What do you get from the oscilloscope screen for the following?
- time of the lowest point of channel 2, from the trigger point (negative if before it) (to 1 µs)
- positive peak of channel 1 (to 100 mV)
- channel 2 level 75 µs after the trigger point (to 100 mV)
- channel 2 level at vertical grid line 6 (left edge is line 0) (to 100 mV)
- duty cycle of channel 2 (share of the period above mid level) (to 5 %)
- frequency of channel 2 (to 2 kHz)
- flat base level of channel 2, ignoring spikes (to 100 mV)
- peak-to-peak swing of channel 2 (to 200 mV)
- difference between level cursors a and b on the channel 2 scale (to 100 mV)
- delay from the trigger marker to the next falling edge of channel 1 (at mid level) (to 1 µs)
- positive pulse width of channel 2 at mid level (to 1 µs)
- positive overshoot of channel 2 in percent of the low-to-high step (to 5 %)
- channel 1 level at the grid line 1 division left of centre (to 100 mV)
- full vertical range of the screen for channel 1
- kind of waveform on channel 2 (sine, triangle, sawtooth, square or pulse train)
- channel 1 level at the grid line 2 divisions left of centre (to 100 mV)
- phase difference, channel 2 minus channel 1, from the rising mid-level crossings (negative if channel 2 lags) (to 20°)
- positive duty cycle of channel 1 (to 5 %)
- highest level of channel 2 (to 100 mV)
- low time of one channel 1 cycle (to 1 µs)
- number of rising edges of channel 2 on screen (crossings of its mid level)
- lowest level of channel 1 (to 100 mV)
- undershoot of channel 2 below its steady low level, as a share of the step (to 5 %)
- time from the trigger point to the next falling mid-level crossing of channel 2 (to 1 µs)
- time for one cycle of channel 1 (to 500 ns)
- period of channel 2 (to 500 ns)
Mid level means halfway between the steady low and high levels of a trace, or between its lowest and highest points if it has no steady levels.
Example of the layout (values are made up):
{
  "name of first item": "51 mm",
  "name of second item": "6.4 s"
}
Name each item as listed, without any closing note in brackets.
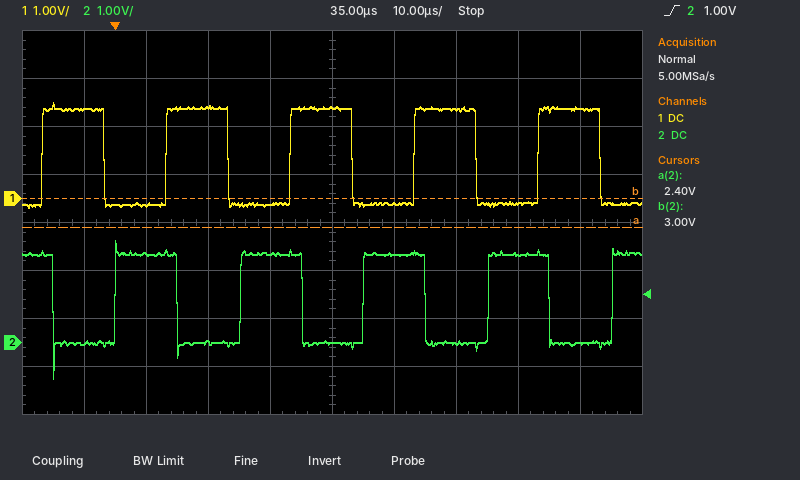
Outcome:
{
  "time of the lowest point of channel 2, from the trigger point (negative if before it)": "-10 µs",
  "positive peak of channel 1": "2.0 V",
  "channel 2 level 75 µs after the trigger point": "0.0 V",
  "channel 2 level at vertical grid line 6 (left edge is line 0)": "1.8 V",
  "duty cycle of channel 2 (share of the period above mid level)": "50 %",
  "frequency of channel 2": "50 kHz",
  "flat base level of channel 2, ignoring spikes": "0.0 V",
  "peak-to-peak swing of channel 2": "2.8 V",
  "difference between level cursors a and b on the channel 2 scale": "600 mV",
  "delay from the trigger marker to the next falling edge of channel 1 (at mid level)": "18 µs",
  "positive pulse width of channel 2 at mid level": "10 µs",
  "positive overshoot of channel 2 in percent of the low-to-high step": "15 %",
  "channel 1 level at the grid line 1 division left of centre": "-100 mV",
  "full vertical range of the screen for channel 1": "8 V",
  "kind of waveform on channel 2": "square",
  "channel 1 level at the grid line 2 divisions left of centre": "1.9 V",
  "phase difference, channel 2 minus channel 1, from the rising mid-level crossings (negative if channel 2 lags)": "+140°",
  "positive duty cycle of channel 1": "50 %",
  "highest level of channel 2": "2.1 V",
  "low time of one channel 1 cycle": "10 µs",
  "number of rising edges of channel 2 on screen": "5",
  "lowest level of channel 1": "-200 mV",
  "undershoot of channel 2 below its steady low level, as a share of the step": "40 %",
  "time from the trigger point to the next falling mid-level crossing of channel 2": "10 µs",
  "time for one cycle of channel 1": "20.0 µs",
  "period of channel 2": "20.0 µs"
}
